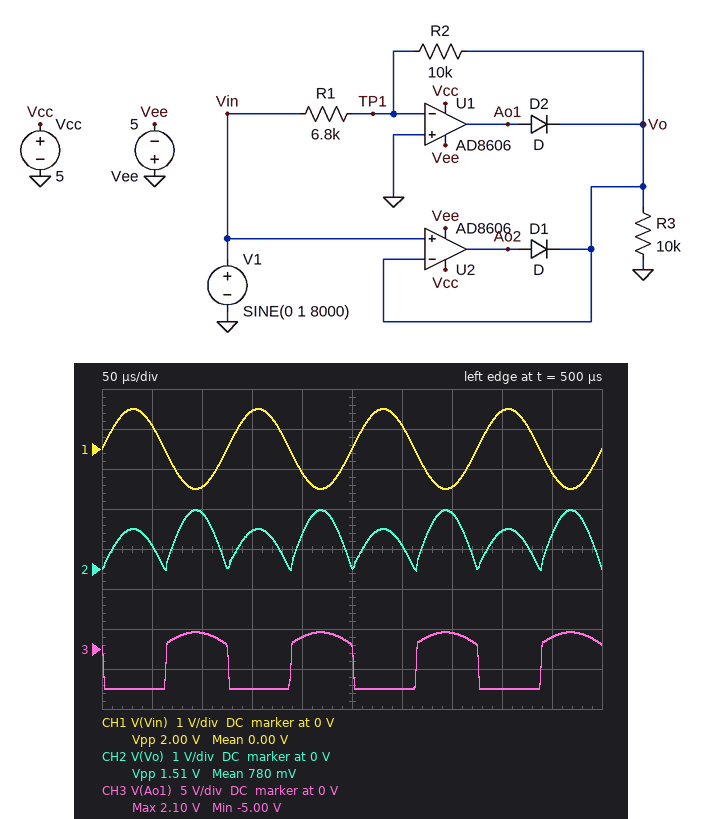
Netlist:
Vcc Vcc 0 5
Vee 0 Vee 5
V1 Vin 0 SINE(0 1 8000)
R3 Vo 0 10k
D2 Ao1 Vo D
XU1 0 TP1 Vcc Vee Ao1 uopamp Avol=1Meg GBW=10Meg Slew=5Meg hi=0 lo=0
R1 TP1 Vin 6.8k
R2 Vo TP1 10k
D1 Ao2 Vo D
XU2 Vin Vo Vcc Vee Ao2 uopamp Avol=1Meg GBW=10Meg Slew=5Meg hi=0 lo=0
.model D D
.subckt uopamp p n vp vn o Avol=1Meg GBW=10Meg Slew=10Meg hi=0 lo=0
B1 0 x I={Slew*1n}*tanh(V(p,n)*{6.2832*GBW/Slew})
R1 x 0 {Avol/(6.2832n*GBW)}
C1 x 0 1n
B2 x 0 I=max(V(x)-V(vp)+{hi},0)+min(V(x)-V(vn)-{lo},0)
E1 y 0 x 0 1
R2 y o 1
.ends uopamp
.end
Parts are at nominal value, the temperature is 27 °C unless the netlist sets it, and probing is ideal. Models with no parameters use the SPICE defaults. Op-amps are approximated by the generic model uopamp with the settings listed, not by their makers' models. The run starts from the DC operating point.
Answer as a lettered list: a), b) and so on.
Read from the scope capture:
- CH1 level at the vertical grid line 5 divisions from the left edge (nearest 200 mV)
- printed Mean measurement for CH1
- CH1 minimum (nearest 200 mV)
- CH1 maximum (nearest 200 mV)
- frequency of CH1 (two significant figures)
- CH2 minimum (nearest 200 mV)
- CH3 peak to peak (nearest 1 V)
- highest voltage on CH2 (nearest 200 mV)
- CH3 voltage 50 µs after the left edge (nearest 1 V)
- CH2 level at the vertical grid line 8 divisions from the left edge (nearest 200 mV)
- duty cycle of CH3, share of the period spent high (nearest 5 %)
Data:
a) 0 V
b) 0.00 V
c) -1.0 V
d) 1.0 V
e) 8.0 kHz
f) 0 V
g) 7 V
h) 1.4 V
i) -5 V
j) 1.0 V
k) 50 %
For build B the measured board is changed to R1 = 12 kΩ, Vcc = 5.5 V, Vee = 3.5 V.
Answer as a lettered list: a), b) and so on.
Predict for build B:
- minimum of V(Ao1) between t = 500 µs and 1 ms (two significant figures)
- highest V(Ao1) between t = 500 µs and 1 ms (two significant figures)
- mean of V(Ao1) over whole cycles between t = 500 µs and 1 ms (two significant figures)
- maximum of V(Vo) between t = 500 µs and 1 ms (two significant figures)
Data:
a) -3.5 V
b) 1.4 V
c) -1.2 V
d) 1.0 V
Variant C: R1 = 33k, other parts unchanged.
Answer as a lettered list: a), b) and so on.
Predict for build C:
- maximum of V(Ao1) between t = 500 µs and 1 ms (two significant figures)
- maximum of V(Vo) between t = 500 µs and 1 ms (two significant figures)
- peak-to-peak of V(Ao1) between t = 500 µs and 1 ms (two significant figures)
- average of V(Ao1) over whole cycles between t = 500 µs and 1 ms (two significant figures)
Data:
a) 890 mV
b) 1.0 V
c) 5.9 V
d) -2.1 V
